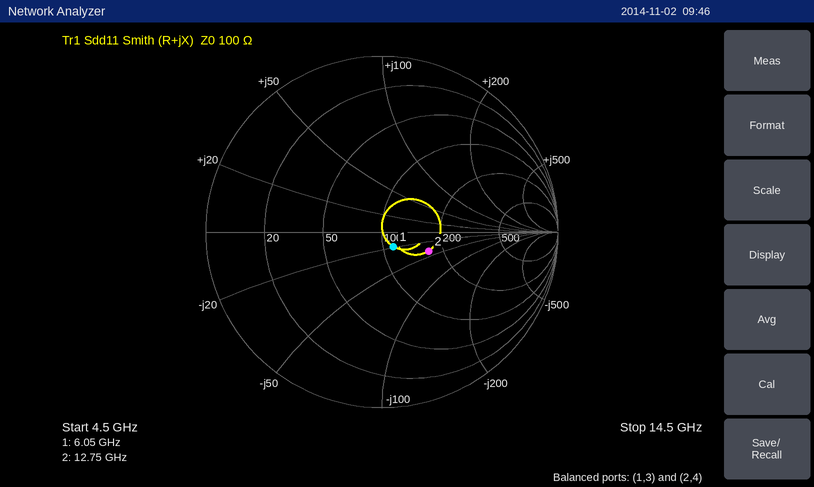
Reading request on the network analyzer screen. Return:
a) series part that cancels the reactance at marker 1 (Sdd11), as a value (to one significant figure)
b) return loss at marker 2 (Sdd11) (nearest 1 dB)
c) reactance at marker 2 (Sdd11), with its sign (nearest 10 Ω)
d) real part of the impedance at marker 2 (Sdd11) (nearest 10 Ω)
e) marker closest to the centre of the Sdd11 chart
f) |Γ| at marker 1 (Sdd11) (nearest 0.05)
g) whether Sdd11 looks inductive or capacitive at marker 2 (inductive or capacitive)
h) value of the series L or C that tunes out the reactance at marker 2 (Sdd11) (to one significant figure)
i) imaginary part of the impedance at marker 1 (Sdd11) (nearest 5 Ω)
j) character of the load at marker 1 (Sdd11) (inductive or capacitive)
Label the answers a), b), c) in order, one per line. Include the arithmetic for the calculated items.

a) L = 20 Ω/(2π × 6.05 GHz) ≈ 526 pH, so 500 pH to one significant figure
b) 11 dB
c) -40 Ω
d) 170 Ω
e) marker 1
f) 0.10
g) capacitive
h) L = 40 Ω/(2π × 12.75 GHz) ≈ 499 pH, so 500 pH to one significant figure
i) -20 Ω
j) capacitive
